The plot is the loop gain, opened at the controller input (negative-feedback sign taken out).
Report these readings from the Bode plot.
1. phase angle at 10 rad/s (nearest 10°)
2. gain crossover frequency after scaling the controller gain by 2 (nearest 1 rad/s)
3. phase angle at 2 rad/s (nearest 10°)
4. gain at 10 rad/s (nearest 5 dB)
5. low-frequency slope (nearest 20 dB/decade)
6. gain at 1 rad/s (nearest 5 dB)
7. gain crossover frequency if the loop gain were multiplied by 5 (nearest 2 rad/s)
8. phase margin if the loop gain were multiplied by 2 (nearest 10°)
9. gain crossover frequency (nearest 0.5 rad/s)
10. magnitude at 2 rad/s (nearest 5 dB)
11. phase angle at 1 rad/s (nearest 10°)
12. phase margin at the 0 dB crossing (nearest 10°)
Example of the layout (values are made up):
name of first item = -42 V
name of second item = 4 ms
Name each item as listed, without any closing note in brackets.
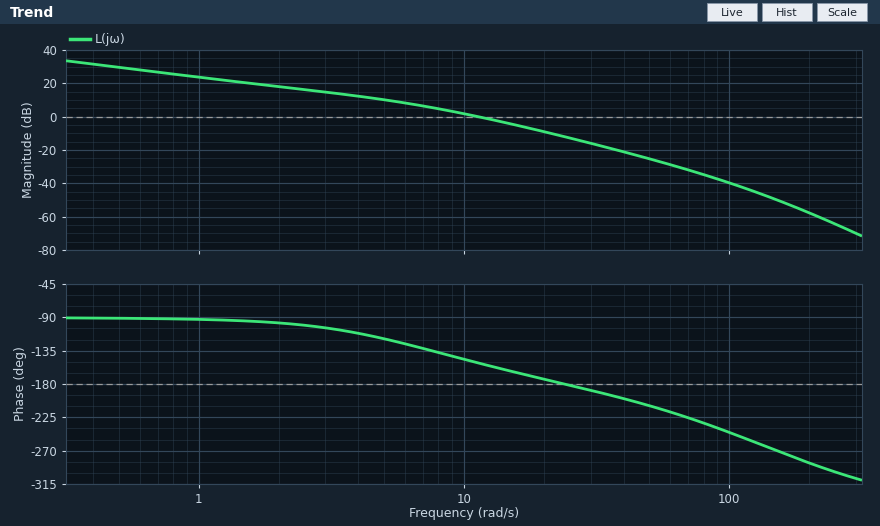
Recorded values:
phase angle at 10 rad/s = -150°
gain crossover frequency after scaling the controller gain by 2 = 17 rad/s
phase angle at 2 rad/s = -100°
gain at 10 rad/s = 0 dB
low-frequency slope = -20 dB/decade
gain at 1 rad/s = 25 dB
gain crossover frequency if the loop gain were multiplied by 5 = 26 rad/s
phase margin if the loop gain were multiplied by 2 = 10°
gain crossover frequency = 11.5 rad/s
magnitude at 2 rad/s = 20 dB
phase angle at 1 rad/s = -90°
phase margin at the 0 dB crossing = 30°
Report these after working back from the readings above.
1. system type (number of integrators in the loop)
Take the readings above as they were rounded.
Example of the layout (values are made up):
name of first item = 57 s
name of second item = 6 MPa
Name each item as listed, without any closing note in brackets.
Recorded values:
system type = 1
